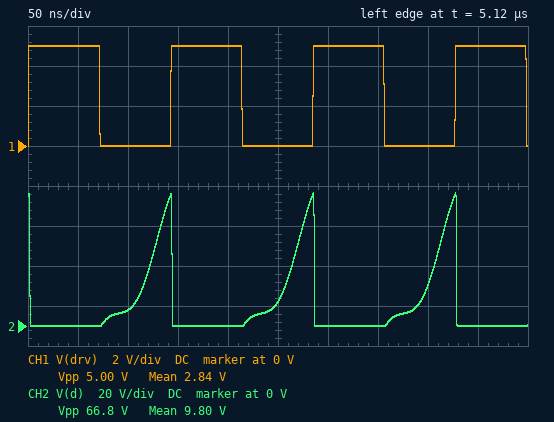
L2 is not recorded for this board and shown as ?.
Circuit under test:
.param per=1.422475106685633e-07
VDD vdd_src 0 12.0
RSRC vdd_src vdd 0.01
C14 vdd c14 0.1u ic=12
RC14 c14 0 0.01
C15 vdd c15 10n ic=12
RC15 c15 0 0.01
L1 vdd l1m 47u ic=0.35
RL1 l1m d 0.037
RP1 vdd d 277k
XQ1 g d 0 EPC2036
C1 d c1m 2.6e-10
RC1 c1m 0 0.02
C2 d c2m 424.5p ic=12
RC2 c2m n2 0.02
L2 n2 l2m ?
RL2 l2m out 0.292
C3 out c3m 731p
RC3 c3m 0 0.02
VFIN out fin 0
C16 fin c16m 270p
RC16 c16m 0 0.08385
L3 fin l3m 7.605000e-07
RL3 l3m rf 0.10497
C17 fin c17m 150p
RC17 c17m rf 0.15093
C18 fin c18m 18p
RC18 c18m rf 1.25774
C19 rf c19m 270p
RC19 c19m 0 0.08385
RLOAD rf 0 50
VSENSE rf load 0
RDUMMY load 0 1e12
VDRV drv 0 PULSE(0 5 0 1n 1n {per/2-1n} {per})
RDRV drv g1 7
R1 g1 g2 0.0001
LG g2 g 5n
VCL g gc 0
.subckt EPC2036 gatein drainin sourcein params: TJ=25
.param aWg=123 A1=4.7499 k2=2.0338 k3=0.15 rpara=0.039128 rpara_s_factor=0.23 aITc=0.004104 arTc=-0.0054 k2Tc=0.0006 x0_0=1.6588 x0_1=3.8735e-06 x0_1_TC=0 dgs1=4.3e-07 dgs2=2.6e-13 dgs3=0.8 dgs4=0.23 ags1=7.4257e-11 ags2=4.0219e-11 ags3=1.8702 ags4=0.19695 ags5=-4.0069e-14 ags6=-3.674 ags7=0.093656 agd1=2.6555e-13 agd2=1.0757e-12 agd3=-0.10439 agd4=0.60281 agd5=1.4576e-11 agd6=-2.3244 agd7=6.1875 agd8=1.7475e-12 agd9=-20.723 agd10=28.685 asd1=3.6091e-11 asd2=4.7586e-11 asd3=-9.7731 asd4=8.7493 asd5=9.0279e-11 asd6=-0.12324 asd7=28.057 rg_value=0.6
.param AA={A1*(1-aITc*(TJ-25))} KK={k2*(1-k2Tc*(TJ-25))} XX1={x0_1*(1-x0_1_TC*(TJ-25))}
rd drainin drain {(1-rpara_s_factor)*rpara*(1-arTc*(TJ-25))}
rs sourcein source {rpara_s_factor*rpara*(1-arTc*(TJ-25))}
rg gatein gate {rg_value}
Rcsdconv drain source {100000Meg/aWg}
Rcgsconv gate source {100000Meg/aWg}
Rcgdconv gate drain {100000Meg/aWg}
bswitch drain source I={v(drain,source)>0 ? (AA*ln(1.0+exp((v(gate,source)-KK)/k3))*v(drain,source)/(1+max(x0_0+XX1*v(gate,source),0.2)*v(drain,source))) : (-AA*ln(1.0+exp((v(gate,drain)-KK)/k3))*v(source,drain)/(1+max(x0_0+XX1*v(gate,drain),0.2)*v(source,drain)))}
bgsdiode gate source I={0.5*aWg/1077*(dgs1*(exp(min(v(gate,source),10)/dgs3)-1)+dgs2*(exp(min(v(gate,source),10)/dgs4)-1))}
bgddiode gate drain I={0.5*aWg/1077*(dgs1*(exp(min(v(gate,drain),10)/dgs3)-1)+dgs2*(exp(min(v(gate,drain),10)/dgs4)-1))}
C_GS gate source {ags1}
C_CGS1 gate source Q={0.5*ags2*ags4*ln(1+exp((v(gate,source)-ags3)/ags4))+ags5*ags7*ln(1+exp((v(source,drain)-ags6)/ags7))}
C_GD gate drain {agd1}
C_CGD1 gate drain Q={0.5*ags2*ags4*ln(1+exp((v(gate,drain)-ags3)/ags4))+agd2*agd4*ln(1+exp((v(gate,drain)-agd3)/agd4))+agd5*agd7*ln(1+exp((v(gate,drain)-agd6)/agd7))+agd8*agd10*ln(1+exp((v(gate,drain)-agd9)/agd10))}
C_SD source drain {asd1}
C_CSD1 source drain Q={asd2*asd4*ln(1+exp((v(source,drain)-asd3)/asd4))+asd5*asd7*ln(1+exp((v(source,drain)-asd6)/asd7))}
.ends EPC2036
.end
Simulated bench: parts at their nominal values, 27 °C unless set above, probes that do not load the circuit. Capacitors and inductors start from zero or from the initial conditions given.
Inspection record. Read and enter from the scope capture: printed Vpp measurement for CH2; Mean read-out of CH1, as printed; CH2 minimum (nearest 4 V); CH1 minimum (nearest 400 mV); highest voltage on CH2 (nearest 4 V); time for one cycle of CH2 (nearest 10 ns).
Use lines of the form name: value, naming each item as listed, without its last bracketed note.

printed Vpp measurement for CH2: 66.8 V
Mean read-out of CH1, as printed: 2.84 V
CH2 minimum: 0 V
CH1 minimum: 0 V
highest voltage on CH2: 68 V
time for one cycle of CH2: 140 ns
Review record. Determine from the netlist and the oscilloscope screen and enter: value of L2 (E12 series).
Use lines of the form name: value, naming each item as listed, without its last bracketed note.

value of L2: 1 µH
